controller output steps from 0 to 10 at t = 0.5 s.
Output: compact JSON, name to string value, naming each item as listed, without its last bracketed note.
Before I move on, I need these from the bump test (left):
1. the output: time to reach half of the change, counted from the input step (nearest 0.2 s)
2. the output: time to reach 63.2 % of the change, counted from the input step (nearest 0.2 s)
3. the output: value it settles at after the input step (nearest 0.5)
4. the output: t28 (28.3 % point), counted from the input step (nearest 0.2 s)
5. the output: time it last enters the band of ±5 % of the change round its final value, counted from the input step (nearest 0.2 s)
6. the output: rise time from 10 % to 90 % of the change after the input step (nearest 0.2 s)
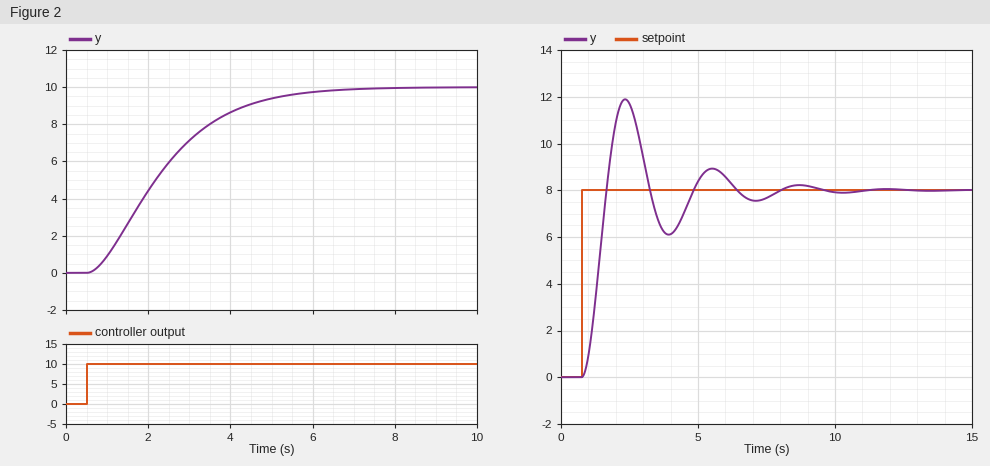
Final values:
{"the output: time to reach half of the change, counted from the input step": "1.6 s", "the output: time to reach 63.2 % of the change, counted from the input step": "2.2 s", "the output: value it settles at after the input step": "10.0", "the output: t28 (28.3 % point), counted from the input step": "1.0 s", "the output: time it last enters the band of ±5 % of the change round its final value, counted from the input step": "4.8 s", "the output: rise time from 10 % to 90 % of the change after the input step": "3.4 s"}
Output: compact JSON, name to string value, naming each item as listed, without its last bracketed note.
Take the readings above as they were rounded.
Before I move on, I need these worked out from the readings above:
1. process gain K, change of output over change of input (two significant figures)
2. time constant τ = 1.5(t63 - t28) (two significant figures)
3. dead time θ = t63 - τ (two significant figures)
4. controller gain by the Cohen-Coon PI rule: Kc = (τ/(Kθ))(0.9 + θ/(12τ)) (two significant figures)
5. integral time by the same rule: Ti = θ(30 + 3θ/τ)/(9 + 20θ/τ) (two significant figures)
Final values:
{"process gain K, change of output over change of input": "1.0", "time constant τ = 1.5(t63 - t28)": "1.8 s", "dead time θ = t63 - τ": "0.40 s", "controller gain by the Cohen-Coon PI rule: Kc = (τ/(Kθ))(0.9 + θ/(12τ))": "4.1", "integral time by the same rule: Ti = θ(30 + 3θ/τ)/(9 + 20θ/τ)": "0.91 s"}
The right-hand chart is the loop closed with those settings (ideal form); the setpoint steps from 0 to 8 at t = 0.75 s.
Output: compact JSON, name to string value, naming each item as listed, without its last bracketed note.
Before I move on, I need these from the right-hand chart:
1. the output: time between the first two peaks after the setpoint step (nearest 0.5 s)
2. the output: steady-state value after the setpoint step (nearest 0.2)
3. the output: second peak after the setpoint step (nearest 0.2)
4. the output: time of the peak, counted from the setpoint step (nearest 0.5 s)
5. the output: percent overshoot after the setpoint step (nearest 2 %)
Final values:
{"the output: time between the first two peaks after the setpoint step": "3.0 s", "the output: steady-state value after the setpoint step": "8.0", "the output: second peak after the setpoint step": "9.0", "the output: time of the peak, counted from the setpoint step": "1.5 s", "the output: percent overshoot after the setpoint step": "48 %"}
